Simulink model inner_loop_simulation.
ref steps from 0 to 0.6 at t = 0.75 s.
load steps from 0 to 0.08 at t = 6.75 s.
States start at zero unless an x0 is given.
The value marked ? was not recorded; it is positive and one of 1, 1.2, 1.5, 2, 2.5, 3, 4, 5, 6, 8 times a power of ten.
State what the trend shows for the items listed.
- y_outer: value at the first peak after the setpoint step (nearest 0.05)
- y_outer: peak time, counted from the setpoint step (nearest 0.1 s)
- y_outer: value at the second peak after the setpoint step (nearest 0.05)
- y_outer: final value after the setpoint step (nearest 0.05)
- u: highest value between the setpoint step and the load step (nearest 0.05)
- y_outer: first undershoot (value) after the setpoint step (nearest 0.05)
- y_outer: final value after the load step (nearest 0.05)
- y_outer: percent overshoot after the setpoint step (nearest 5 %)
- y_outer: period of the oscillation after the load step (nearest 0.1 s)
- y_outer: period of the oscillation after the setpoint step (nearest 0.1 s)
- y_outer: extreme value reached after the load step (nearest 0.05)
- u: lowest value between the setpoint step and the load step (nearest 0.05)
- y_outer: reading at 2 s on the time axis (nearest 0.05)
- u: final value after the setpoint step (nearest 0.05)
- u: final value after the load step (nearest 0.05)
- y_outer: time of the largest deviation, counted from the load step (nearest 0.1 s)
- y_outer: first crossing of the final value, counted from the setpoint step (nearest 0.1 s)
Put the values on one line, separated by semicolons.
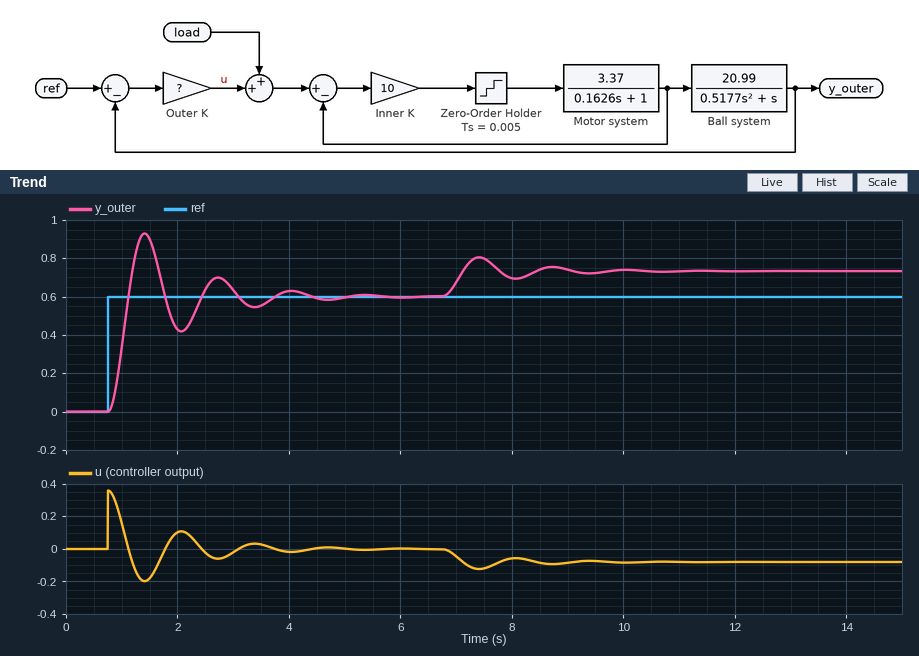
0.95; 0.7 s; 0.70; 0.60; 0.35; 0.40; 0.75; 55 %; 1.3 s; 1.3 s; 0.80; -0.20; 0.45; 0.00; -0.10; 0.7 s; 0.4 s
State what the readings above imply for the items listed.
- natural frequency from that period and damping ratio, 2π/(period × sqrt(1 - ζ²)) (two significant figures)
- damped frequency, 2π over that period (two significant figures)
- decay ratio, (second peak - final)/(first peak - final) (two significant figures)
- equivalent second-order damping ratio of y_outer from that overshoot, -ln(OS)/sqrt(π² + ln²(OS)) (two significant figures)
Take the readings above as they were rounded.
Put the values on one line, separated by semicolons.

4.9 rad/s; 4.8 rad/s; 0.29; 0.19
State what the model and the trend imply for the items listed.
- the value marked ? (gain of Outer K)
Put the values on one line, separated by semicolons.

0.6
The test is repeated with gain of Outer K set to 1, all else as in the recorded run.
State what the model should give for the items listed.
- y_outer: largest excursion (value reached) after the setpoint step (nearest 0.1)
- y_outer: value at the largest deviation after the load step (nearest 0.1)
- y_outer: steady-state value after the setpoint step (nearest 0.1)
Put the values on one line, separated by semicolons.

1.0; 0.7; 0.6
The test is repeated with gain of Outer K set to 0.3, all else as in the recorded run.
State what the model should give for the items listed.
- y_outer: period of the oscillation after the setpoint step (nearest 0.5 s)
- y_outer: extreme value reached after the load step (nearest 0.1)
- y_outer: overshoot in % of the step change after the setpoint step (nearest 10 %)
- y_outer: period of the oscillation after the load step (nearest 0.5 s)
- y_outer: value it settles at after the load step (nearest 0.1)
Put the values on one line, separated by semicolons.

2.0 s; 1.0; 40 %; 2.0 s; 0.9
